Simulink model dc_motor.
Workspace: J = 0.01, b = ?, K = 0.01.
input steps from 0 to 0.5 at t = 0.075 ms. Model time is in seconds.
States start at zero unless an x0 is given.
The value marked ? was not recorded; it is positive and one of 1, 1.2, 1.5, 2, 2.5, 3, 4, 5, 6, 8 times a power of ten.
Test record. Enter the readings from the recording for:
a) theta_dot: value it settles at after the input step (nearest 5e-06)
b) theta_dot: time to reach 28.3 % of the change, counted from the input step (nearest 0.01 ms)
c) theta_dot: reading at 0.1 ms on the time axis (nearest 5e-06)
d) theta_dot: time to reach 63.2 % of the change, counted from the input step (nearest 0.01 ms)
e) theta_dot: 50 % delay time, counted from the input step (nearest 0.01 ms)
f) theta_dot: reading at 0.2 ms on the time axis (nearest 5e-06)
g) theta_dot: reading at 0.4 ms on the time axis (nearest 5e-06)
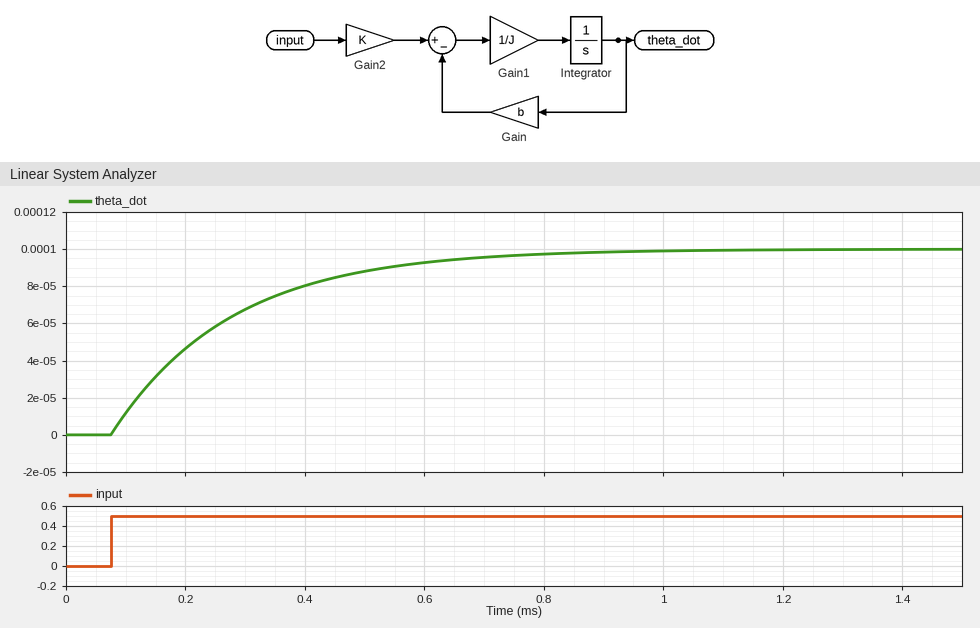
0.000100
0.07 ms
0.000010
0.20 ms
0.14 ms
0.000045
0.000080
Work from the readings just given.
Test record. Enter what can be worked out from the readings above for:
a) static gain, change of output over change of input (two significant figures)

0.00020
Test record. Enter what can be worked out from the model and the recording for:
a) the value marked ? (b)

50
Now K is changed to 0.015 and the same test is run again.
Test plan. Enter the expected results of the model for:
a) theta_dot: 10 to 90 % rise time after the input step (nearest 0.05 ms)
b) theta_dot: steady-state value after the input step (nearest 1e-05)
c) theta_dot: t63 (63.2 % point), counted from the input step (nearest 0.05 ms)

0.45 ms
0.00015
0.20 ms
